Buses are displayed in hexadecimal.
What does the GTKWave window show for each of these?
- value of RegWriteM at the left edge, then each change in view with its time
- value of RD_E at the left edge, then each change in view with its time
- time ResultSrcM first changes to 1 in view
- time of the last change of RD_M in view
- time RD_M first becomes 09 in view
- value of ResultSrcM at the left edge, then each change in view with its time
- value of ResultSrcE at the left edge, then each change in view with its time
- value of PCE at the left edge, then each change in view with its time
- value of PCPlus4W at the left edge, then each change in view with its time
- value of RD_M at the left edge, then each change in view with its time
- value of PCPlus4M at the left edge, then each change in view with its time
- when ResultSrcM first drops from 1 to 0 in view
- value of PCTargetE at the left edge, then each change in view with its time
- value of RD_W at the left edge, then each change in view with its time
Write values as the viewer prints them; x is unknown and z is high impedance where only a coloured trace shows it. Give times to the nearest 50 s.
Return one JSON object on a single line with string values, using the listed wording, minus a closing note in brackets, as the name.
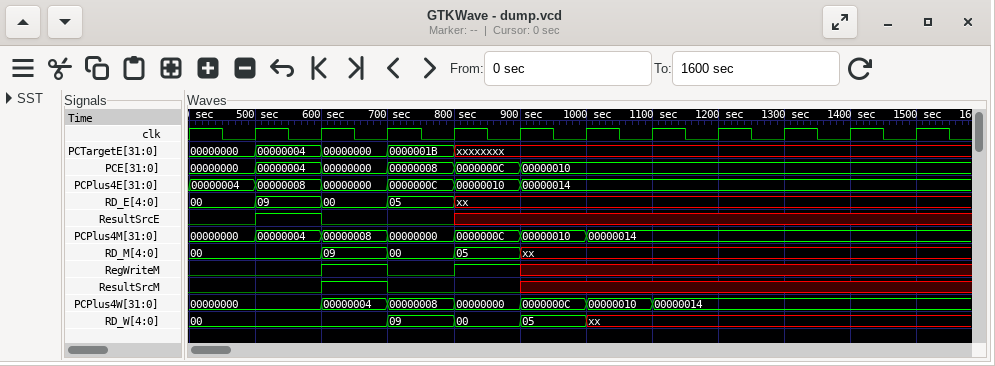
{"value of RegWriteM at the left edge, then each change in view with its time": "0, 1 at 600 s, 0 at 700 s, 1 at 800 s, x at 900 s", "value of RD_E at the left edge, then each change in view with its time": "00, 09 at 500 s, 00 at 600 s, 05 at 700 s, xx at 800 s", "time ResultSrcM first changes to 1 in view": "600 s", "time of the last change of RD_M in view": "900 s", "time RD_M first becomes 09 in view": "600 s", "value of ResultSrcM at the left edge, then each change in view with its time": "0, 1 at 600 s, 0 at 700 s, x at 900 s", "value of ResultSrcE at the left edge, then each change in view with its time": "0, 1 at 500 s, 0 at 600 s, x at 800 s", "value of PCE at the left edge, then each change in view with its time": "00000000, 00000004 at 500 s, 00000000 at 600 s, 00000008 at 700 s, 0000000C at 800 s, 00000010 at 900 s", "value of PCPlus4W at the left edge, then each change in view with its time": "00000000, 00000004 at 600 s, 00000008 at 700 s, 00000000 at 800 s, 0000000C at 900 s, 00000010 at 1000 s, 00000014 at 1100 s", "value of RD_M at the left edge, then each change in view with its time": "00, 09 at 600 s, 00 at 700 s, 05 at 800 s, xx at 900 s", "value of PCPlus4M at the left edge, then each change in view with its time": "00000000, 00000004 at 500 s, 00000008 at 600 s, 00000000 at 700 s, 0000000C at 800 s, 00000010 at 900 s, 00000014 at 1000 s", "when ResultSrcM first drops from 1 to 0 in view": "700 s", "value of PCTargetE at the left edge, then each change in view with its time": "00000000, 00000004 at 500 s, 00000000 at 600 s, 0000001B at 700 s, xxxxxxxx at 800 s", "value of RD_W at the left edge, then each change in view with its time": "00, 09 at 700 s, 00 at 800 s, 05 at 900 s, xx at 1000 s"}
